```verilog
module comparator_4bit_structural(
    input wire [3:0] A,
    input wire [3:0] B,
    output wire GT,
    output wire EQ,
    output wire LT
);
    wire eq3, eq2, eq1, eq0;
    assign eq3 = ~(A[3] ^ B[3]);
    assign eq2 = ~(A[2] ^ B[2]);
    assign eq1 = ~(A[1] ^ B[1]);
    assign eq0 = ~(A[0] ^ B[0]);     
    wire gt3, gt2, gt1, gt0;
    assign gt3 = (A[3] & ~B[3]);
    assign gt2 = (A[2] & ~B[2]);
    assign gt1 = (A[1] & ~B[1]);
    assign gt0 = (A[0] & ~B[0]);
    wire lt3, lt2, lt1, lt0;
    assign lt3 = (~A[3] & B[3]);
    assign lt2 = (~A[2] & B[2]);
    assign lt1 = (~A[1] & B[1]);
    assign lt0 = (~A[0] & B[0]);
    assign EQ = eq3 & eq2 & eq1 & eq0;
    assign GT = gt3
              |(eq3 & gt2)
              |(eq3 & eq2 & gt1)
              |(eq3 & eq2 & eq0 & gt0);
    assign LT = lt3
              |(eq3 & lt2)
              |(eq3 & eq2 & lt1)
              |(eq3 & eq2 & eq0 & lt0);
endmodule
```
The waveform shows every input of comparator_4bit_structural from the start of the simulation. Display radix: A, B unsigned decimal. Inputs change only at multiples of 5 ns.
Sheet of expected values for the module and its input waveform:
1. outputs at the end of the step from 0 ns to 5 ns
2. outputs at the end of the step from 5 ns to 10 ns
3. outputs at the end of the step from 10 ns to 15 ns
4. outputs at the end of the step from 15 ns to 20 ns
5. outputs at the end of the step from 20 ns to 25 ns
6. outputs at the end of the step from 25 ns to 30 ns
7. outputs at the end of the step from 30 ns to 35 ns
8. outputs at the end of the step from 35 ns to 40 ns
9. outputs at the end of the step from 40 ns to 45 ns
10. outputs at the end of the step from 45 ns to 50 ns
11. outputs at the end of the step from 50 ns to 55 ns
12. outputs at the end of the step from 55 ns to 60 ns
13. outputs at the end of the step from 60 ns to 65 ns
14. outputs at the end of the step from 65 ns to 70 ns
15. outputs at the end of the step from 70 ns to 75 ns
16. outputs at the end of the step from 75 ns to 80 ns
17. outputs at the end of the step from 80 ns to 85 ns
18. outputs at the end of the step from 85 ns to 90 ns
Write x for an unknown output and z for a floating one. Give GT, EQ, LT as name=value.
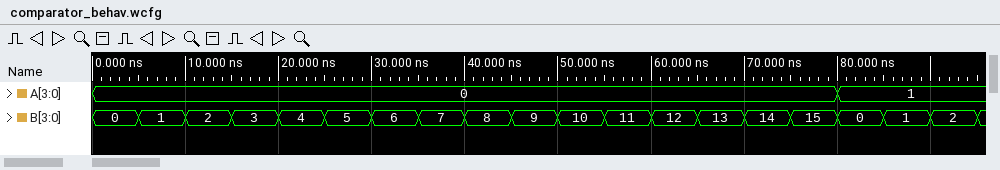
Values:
GT=0, EQ=1, LT=0
GT=0, EQ=0, LT=0
GT=0, EQ=0, LT=1
GT=0, EQ=0, LT=1
GT=0, EQ=0, LT=1
GT=0, EQ=0, LT=1
GT=0, EQ=0, LT=1
GT=0, EQ=0, LT=1
GT=0, EQ=0, LT=1
GT=0, EQ=0, LT=1
GT=0, EQ=0, LT=1
GT=0, EQ=0, LT=1
GT=0, EQ=0, LT=1
GT=0, EQ=0, LT=1
GT=0, EQ=0, LT=1
GT=0, EQ=0, LT=1
GT=0, EQ=0, LT=0
GT=0, EQ=1, LT=0
